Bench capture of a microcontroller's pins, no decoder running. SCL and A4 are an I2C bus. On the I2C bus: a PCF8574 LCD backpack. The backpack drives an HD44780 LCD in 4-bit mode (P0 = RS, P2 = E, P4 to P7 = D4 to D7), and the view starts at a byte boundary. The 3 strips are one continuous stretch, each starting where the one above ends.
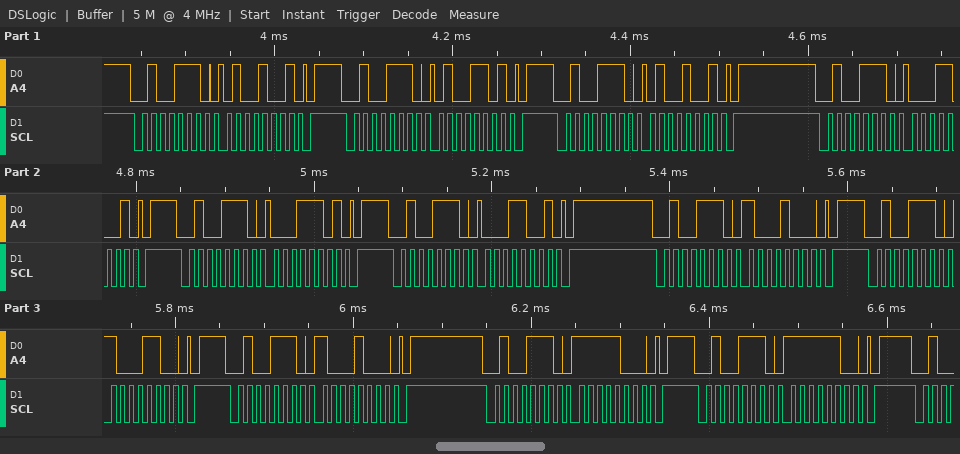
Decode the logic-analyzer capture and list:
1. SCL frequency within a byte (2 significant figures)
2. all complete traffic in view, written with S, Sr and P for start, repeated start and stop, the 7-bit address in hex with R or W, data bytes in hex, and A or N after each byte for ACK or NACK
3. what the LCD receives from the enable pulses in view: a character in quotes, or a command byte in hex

100 kHz
S 27W A 49 A P S 27W A 4D A P S 27W A 49 A P S 27W A 19 A P S 27W A 1D A P S 27W A 19 A P S 27W A 88 A P S 27W A 8C A P S 27W A 88 A P S 27W A F8 A P S 27W A FC A P
'A'
